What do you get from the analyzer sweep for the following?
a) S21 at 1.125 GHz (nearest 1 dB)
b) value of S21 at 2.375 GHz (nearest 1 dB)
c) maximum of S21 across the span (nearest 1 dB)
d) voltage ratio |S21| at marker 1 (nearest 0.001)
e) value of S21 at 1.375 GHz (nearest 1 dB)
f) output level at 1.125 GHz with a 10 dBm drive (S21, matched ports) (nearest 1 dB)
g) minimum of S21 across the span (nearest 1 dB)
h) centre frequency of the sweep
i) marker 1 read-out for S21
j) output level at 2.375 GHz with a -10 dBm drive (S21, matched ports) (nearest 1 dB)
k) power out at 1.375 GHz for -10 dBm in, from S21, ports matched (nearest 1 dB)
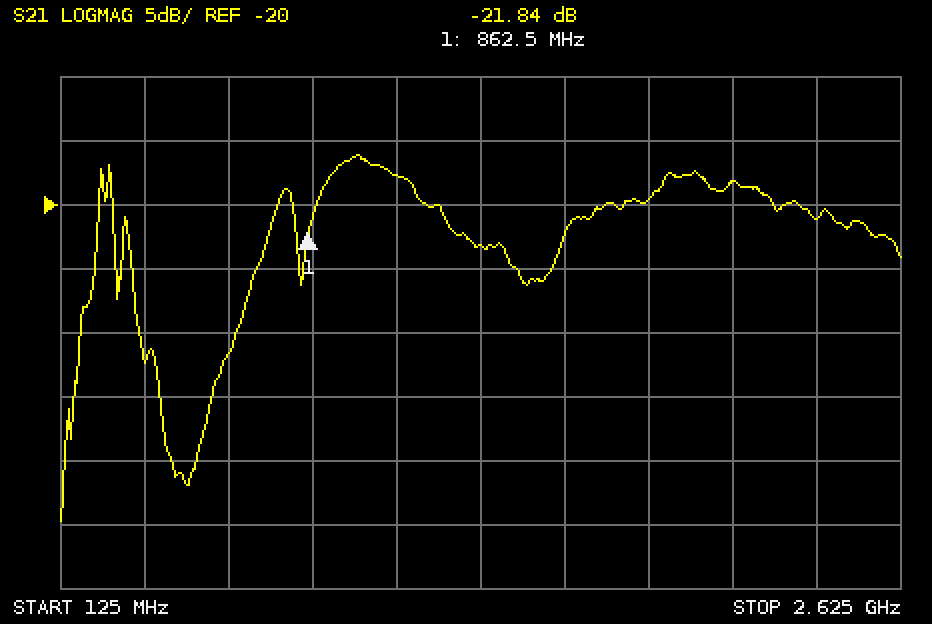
-18 dB
-21 dB
-16 dB
0.081
-23 dB
-8 dBm
-45 dB
1.375 GHz
-21.84 dB
-31 dBm
-33 dBm
